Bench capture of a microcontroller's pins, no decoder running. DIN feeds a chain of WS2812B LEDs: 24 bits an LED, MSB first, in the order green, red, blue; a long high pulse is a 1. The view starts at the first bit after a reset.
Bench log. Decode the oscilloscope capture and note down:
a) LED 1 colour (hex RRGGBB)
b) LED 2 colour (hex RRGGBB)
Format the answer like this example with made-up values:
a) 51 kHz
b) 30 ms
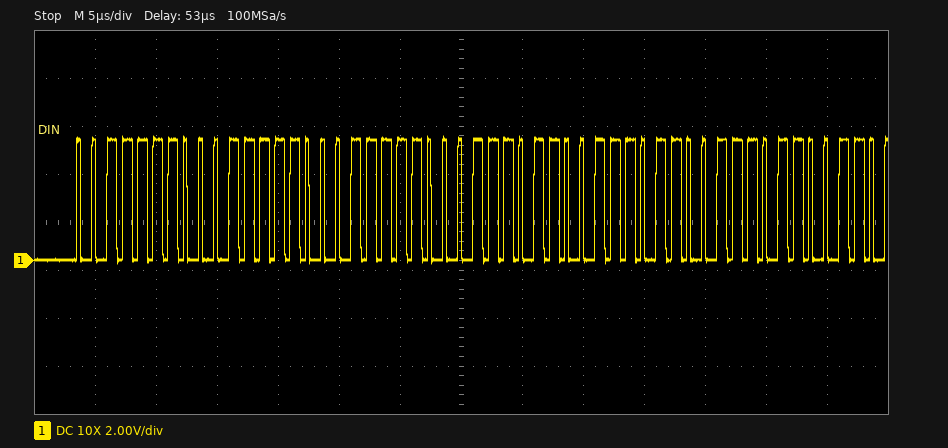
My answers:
a) #3E3E3E
b) #3B3B3B
